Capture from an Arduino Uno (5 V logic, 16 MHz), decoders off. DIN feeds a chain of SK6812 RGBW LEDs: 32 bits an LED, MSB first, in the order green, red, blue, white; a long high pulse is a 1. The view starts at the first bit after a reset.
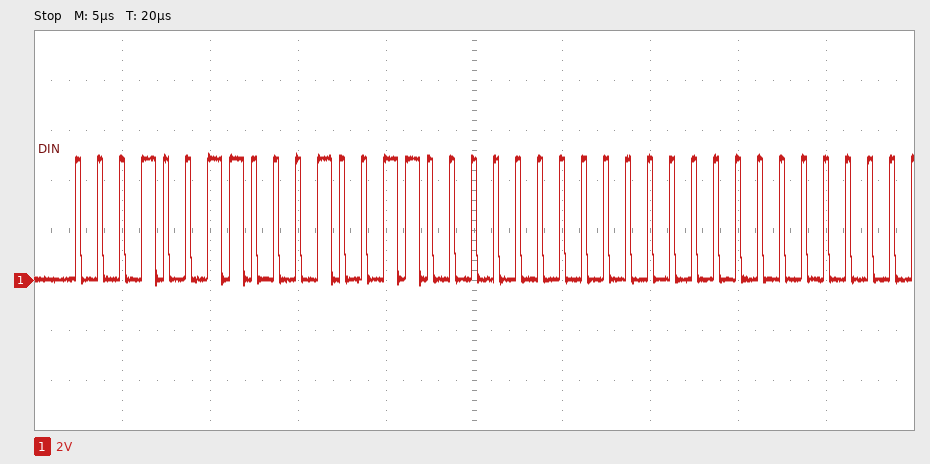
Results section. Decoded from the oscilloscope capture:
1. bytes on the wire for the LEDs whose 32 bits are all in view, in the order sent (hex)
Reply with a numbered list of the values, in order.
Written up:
1. 13 13 00 00
